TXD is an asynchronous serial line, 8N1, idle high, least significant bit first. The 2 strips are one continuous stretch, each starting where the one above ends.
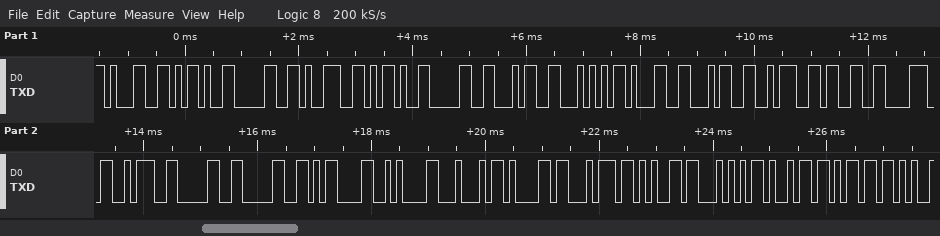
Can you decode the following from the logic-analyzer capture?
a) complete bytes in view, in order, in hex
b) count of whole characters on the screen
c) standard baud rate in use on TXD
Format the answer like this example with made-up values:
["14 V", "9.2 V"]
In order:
["31 2D 30 39 2D 30 34 54 31 34 3A 33 38 3A 30 30 0D 0A 44 61 74 65 54 69 6D", "25", "9600 baud"]
